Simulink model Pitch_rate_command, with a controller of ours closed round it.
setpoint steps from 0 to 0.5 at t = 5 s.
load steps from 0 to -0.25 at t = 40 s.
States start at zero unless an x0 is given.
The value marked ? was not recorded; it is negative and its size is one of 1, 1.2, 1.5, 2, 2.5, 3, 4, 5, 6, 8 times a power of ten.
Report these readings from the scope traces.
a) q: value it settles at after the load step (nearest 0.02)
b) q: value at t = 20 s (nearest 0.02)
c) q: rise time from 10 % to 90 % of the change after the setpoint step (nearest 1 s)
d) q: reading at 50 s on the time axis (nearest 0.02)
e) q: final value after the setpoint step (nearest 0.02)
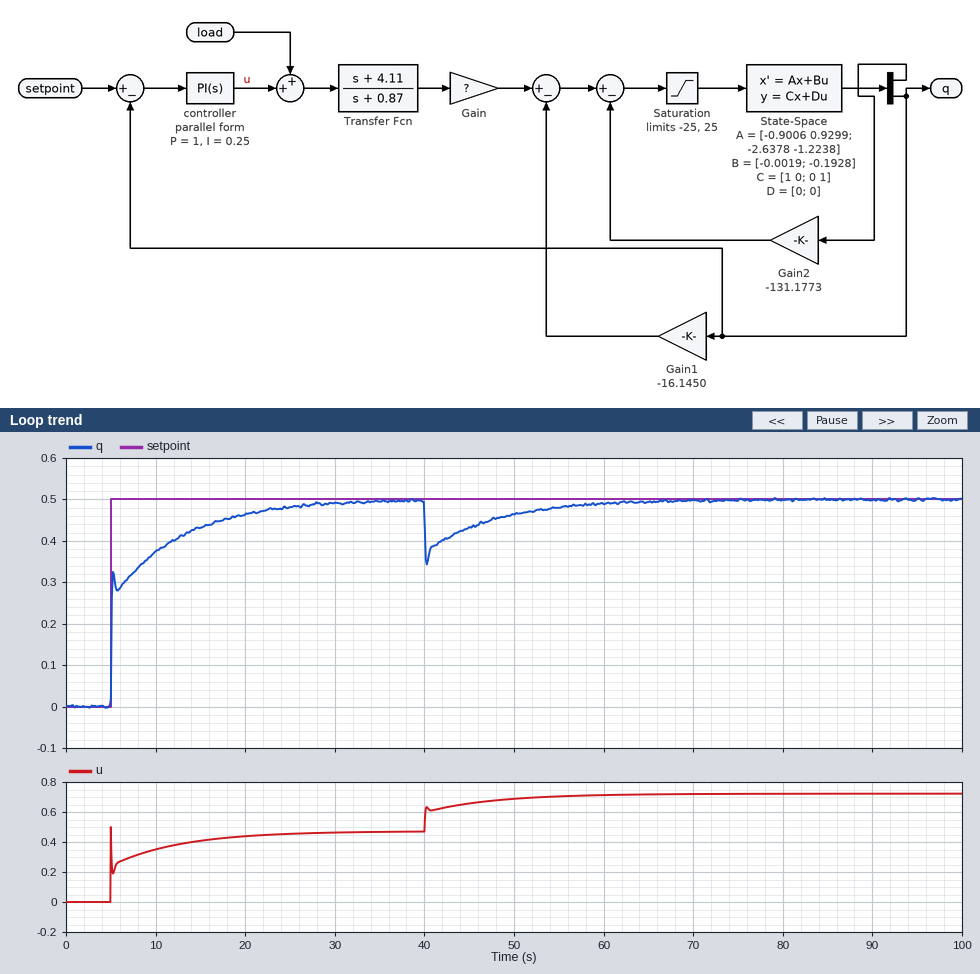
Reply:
0.50
0.46
12 s
0.46
0.50
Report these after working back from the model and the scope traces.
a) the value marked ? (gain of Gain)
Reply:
-40
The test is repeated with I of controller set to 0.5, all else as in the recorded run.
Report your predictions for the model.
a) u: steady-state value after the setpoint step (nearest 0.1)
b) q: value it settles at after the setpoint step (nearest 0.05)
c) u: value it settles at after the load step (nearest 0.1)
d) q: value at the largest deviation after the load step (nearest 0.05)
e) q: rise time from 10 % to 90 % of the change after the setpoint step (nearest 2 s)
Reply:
0.5
0.50
0.7
0.35
6 s
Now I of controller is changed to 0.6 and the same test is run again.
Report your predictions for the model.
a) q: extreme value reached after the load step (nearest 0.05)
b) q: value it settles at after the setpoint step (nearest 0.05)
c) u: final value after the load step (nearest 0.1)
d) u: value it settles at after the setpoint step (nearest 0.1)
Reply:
0.35
0.50
0.7
0.5
